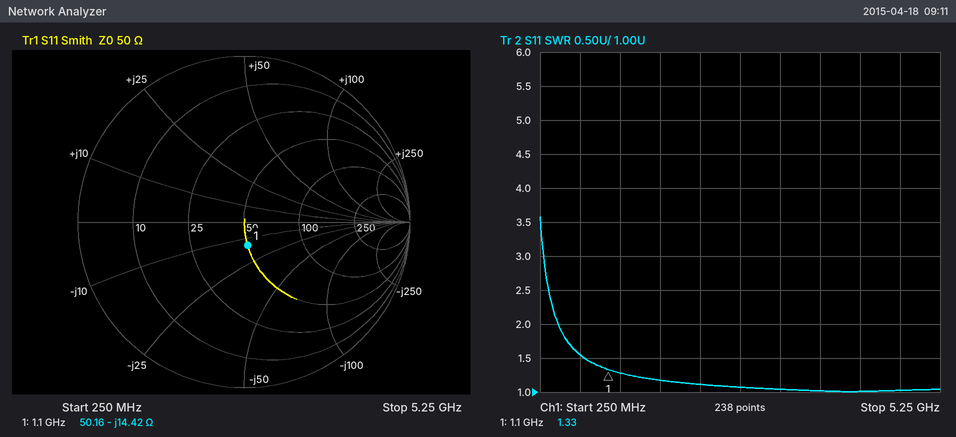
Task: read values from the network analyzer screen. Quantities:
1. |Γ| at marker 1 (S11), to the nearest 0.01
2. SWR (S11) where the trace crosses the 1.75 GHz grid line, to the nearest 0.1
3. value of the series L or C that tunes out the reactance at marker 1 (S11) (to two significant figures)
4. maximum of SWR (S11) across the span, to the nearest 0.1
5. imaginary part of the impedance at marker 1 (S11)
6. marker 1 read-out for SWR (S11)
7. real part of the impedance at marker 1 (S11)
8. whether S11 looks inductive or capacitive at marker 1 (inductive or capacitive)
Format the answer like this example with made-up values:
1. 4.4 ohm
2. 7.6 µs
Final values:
1. 0.14
2. 1.2
3. 2.1 nH
4. 3.6
5. -14.42 Ω
6. 1.33
7. 50.16 Ω
8. capacitive
